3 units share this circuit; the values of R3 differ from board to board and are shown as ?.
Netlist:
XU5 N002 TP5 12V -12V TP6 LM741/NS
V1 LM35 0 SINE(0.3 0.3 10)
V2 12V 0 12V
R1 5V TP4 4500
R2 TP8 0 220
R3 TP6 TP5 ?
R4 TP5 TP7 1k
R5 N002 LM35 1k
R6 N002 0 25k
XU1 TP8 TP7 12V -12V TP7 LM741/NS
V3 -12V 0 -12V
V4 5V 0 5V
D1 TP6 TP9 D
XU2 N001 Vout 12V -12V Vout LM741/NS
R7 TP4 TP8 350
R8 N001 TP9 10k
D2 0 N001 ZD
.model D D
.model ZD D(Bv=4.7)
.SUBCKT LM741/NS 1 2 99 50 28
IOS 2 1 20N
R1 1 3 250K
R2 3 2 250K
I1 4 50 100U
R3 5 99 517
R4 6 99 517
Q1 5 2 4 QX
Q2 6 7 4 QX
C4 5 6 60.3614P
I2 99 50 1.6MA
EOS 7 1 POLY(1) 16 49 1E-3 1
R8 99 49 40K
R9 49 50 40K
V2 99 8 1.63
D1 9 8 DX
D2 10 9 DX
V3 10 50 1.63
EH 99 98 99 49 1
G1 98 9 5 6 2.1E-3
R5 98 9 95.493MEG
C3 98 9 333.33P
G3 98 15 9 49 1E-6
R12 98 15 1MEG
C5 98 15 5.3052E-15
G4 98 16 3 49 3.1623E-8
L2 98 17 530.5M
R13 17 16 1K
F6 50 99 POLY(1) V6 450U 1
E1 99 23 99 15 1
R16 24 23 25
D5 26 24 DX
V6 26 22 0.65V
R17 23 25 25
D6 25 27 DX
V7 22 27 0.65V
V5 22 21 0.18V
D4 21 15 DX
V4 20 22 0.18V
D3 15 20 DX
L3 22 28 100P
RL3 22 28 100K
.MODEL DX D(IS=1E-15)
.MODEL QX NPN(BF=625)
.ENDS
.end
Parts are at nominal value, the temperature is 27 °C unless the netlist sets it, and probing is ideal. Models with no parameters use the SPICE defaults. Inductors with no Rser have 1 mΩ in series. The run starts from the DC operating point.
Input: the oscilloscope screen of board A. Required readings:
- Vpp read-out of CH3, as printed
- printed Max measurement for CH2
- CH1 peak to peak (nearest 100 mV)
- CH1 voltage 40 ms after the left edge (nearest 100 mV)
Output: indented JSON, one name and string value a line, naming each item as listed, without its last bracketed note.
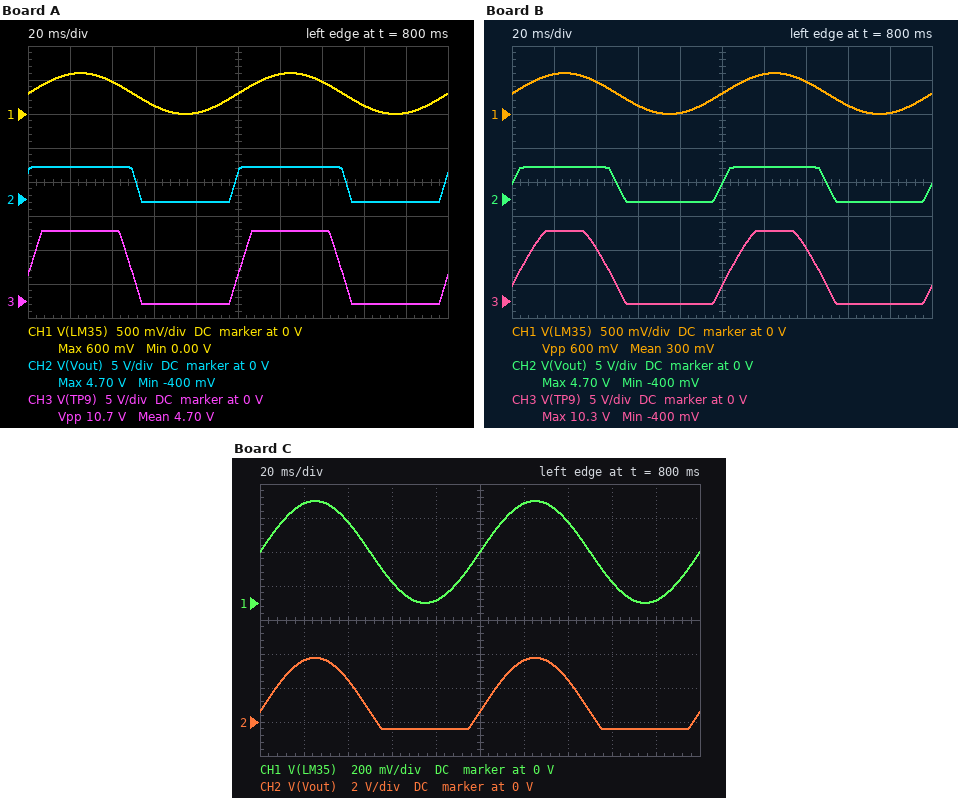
{
  "Vpp read-out of CH3, as printed": "10.7 V",
  "printed Max measurement for CH2": "4.70 V",
  "CH1 peak to peak": "600 mV",
  "CH1 voltage 40 ms after the left edge": "500 mV"
}
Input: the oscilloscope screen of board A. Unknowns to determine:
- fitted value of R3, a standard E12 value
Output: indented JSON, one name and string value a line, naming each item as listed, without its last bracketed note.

{
  "fitted value of R3, a standard E12 value": "56 kΩ"
}
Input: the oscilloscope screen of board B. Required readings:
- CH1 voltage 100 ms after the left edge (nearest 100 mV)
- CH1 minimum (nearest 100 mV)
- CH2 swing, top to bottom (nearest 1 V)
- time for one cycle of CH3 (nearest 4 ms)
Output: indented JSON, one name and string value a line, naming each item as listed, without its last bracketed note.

{
  "CH1 voltage 100 ms after the left edge": "300 mV",
  "CH1 minimum": "0 V",
  "CH2 swing, top to bottom": "5 V",
  "time for one cycle of CH3": "100 ms"
}
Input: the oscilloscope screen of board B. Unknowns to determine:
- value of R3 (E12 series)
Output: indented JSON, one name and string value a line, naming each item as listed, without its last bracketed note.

{
  "value of R3": "33 kΩ"
}
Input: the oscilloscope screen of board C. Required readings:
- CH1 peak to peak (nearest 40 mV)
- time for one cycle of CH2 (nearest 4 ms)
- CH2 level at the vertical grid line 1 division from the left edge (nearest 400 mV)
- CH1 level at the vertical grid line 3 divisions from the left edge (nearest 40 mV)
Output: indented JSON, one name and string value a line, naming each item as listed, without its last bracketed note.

{
  "CH1 peak to peak": "600 mV",
  "time for one cycle of CH2": "100 ms",
  "CH2 level at the vertical grid line 1 division from the left edge": "3.6 V",
  "CH1 level at the vertical grid line 3 divisions from the left edge": "120 mV"
}
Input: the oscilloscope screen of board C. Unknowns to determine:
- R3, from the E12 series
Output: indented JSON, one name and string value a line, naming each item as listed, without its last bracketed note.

{
  "R3, from the E12 series": "10 kΩ"
}
